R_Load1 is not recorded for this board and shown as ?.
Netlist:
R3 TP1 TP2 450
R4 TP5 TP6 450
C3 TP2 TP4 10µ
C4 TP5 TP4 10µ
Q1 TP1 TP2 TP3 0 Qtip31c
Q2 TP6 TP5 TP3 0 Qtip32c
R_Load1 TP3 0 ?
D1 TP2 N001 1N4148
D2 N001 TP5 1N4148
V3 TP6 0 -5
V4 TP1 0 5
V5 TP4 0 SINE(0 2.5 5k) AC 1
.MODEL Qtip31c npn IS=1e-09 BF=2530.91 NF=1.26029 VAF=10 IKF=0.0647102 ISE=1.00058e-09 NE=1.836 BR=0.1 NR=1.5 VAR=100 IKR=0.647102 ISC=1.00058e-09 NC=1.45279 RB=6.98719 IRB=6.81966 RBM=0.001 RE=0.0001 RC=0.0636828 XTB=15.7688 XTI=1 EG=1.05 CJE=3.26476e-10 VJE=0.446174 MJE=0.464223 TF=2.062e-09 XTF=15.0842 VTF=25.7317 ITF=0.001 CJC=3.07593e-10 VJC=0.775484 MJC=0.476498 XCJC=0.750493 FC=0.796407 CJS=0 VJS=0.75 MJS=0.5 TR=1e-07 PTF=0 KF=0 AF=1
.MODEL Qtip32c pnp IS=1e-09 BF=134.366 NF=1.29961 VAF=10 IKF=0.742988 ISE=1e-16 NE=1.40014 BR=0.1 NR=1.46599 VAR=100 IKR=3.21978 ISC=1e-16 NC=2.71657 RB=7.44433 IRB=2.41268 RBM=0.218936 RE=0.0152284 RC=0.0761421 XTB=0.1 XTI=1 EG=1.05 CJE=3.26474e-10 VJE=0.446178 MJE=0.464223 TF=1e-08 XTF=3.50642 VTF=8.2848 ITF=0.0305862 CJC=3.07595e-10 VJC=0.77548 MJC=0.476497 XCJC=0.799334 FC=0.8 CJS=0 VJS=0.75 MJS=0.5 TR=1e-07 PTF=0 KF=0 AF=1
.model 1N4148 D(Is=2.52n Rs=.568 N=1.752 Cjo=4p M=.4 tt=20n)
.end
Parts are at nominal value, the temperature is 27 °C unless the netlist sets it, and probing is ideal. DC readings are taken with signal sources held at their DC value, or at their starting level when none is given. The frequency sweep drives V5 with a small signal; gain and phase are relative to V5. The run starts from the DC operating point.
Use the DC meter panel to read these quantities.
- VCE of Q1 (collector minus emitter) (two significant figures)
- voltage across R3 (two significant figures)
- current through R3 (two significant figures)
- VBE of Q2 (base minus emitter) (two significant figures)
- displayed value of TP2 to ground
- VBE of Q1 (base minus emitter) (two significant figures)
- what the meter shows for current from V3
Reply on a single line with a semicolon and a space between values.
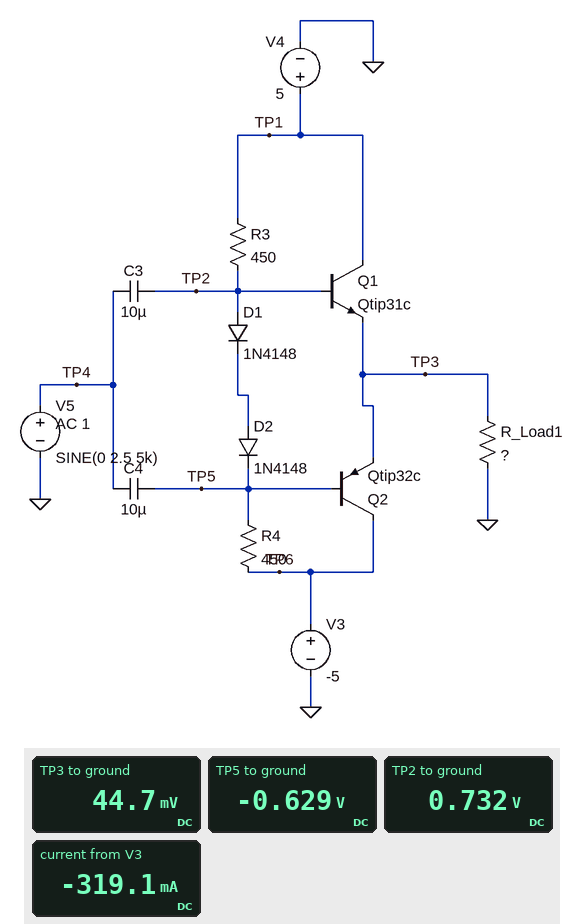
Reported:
5.0 V; 4.3 V; 9.5 mA; -670 mV; 0.732 V; 690 mV; -319.1 mA
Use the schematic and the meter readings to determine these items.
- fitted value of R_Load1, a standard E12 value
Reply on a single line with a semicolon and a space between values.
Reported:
22 Ω
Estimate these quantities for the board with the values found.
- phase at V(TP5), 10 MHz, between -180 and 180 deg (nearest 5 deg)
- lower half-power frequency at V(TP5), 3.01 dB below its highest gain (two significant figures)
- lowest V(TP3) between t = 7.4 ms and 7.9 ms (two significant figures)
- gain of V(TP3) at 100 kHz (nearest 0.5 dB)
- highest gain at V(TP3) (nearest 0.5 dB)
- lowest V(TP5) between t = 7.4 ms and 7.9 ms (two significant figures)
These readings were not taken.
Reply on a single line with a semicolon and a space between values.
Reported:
0 deg; 41 Hz; -2.4 V; 0 dB; 0 dB; -3.1 V
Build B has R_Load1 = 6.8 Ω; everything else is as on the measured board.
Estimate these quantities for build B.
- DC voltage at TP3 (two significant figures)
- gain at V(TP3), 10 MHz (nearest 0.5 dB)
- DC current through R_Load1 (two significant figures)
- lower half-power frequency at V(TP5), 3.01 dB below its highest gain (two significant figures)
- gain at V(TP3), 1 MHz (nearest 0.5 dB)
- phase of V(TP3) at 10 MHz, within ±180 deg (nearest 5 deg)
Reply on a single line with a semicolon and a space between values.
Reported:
38 mV; -3.5 dB; 5.6 mA; 47 Hz; -0.5 dB; -10 deg
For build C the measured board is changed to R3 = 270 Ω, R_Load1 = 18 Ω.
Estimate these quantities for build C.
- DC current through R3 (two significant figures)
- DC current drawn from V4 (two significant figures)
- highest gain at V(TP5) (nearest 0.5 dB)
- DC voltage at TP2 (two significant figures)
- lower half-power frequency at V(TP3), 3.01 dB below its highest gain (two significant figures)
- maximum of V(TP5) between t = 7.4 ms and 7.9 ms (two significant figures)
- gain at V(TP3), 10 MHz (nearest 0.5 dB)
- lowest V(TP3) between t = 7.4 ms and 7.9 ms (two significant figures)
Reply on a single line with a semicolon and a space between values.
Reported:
12 mA; 400 mA; 0 dB; 1.7 V; 54 Hz; 2.8 V; -2.0 dB; -1.5 V
